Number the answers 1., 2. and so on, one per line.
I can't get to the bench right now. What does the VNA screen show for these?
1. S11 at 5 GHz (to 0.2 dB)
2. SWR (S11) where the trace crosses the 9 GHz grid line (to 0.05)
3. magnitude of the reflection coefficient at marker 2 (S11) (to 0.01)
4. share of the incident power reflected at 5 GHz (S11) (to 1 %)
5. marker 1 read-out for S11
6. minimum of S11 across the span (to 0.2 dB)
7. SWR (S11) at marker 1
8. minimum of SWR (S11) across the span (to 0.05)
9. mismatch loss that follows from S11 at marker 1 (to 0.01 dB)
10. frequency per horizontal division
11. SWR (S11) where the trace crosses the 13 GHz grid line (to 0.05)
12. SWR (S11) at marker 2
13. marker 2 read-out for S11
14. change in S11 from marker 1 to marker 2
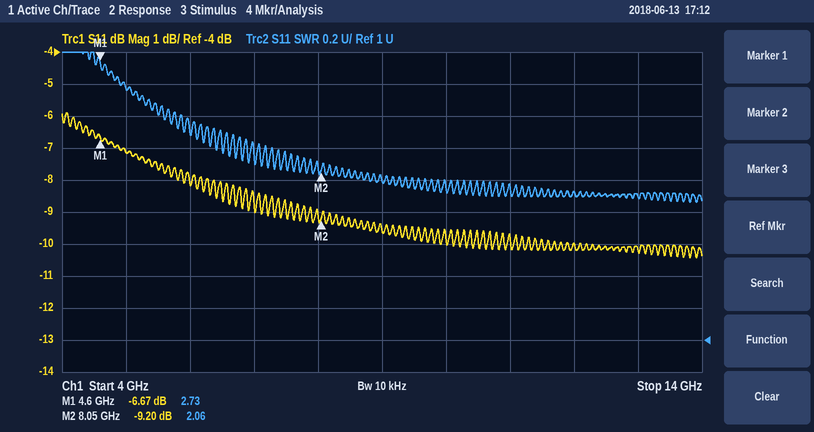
1. -7.2 dB
2. 2.00
3. 0.35
4. 19 %
5. -6.67 dB
6. -10.4 dB
7. 2.73
8. 1.85
9. 1.05 dB
10. 1 GHz
11. 1.90
12. 2.06
13. -9.20 dB
14. -2.53 dB
